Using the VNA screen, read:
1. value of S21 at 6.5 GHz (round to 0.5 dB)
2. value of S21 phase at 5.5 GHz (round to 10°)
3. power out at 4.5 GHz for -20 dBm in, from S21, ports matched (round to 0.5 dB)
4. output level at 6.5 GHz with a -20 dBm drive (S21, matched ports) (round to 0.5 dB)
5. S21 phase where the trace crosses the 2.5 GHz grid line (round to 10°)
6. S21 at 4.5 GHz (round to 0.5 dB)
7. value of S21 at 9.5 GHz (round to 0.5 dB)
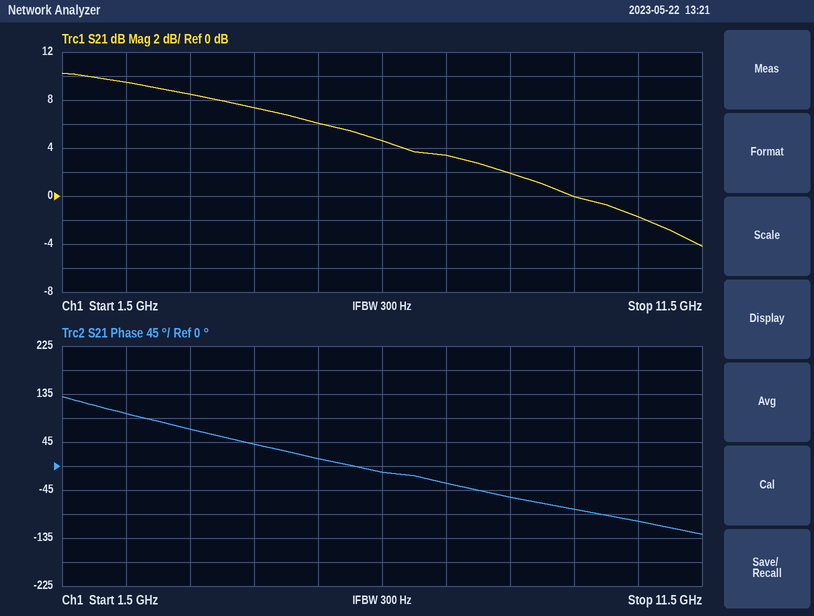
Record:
4.5 dB
10°
-12.5 dBm
-15.5 dBm
100°
7.5 dB
0.0 dB
